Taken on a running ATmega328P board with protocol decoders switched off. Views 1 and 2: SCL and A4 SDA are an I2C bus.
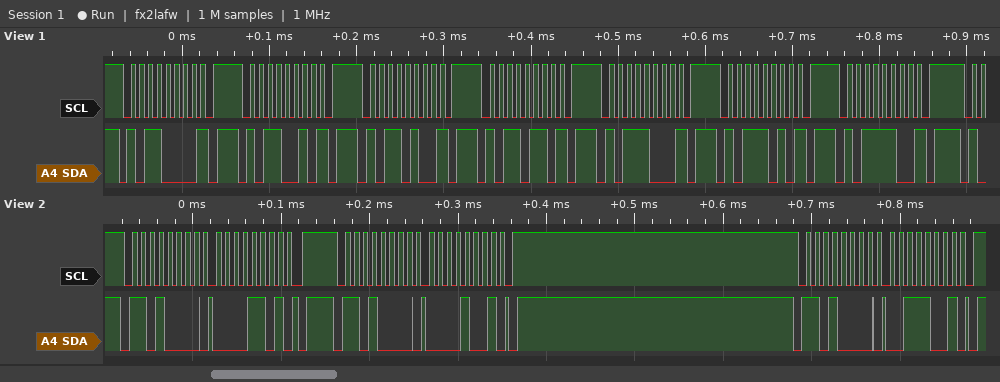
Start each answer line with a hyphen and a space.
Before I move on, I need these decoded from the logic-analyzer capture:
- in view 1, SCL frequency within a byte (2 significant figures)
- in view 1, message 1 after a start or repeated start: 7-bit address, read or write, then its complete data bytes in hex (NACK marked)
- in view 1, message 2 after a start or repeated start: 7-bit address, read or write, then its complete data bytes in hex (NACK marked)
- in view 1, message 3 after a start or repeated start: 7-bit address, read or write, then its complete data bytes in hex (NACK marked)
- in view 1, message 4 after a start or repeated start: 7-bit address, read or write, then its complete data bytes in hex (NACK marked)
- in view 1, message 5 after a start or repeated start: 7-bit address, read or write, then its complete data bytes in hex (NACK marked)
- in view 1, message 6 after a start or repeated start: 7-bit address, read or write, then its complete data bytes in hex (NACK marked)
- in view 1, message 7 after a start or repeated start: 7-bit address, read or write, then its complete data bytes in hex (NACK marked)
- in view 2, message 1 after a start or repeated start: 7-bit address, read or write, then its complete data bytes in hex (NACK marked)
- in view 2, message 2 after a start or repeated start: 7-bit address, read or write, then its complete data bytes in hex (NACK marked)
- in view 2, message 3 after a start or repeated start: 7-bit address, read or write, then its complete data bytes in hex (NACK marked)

- 100 kHz
- 0x58 write NACK
- 0x59 write NACK
- 0x5A write NACK
- 0x5B write NACK
- 0x5C write NACK
- 0x5D write NACK
- 0x5E write NACK
- 0x68 write: 0D
- 0x68 write: 09
- 0x68 write: 39
